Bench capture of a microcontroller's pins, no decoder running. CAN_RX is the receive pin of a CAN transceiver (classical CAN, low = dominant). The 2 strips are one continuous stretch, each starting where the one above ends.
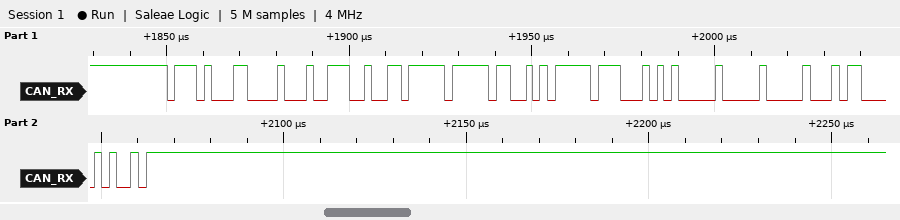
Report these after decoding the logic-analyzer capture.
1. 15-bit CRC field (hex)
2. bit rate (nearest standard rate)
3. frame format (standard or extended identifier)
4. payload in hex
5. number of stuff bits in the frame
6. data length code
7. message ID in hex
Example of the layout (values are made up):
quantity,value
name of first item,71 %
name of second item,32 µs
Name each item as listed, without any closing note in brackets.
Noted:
quantity,value
15-bit CRC field,0x1614
bit rate,500 kbit/s
frame format,standard
payload in hex,9C 9B FF CA FF 15 00 00
number of stuff bits in the frame,6
data length code,8
message ID in hex,0x746
